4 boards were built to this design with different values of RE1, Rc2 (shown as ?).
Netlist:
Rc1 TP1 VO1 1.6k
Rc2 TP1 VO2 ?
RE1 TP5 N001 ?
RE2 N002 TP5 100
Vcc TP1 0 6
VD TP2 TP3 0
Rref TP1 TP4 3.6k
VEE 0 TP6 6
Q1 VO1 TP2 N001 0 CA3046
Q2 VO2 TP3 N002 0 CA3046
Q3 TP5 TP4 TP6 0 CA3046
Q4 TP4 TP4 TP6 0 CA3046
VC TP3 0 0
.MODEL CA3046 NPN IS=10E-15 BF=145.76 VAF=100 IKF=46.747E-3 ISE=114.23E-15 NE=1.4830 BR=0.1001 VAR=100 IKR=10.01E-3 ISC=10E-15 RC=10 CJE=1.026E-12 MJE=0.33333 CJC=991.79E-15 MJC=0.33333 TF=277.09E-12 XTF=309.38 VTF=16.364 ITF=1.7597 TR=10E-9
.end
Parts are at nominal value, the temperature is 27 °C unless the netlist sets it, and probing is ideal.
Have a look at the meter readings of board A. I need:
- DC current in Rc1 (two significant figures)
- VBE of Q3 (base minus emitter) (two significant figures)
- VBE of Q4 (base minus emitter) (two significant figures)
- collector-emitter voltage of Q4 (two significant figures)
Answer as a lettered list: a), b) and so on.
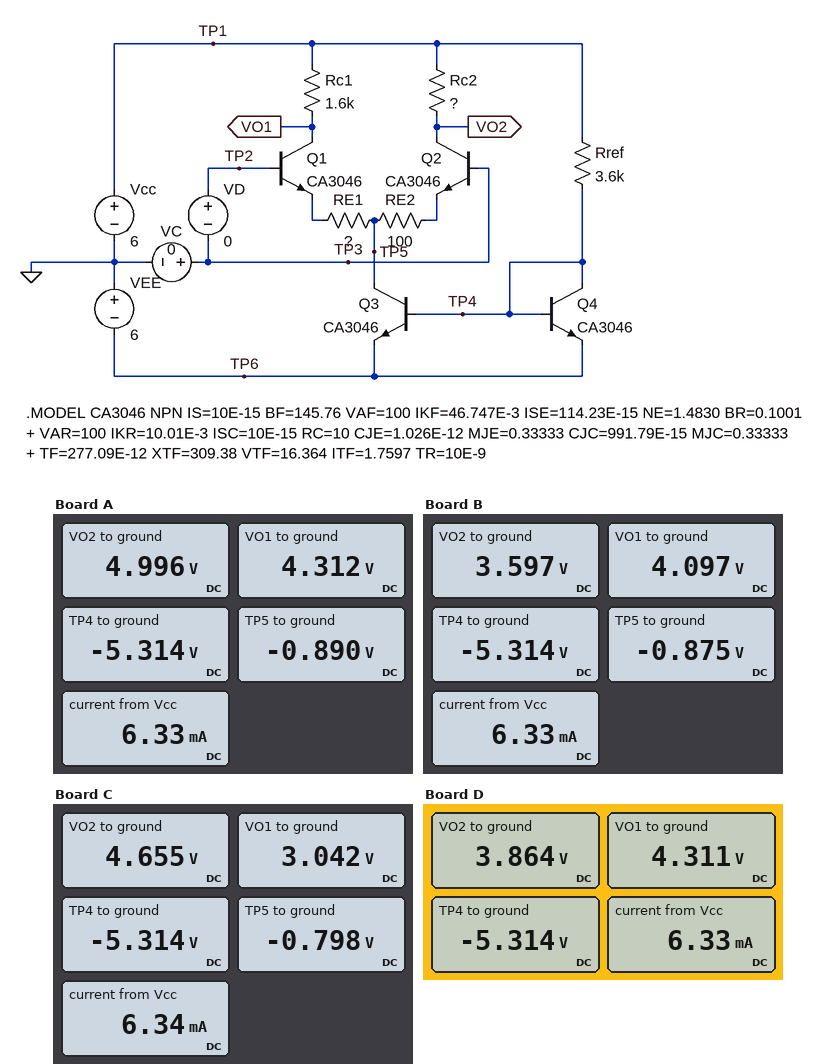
a) 1.1 mA
b) 690 mV
c) 690 mV
d) 690 mV
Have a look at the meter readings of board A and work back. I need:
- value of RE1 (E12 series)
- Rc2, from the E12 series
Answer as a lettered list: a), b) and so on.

a) 220 Ω
b) 470 Ω
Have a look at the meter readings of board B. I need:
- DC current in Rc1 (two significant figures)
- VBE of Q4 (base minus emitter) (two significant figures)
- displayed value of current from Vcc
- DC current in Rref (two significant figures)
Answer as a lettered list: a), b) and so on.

a) 1.2 mA
b) 690 mV
c) 6.33 mA
d) 3.1 mA
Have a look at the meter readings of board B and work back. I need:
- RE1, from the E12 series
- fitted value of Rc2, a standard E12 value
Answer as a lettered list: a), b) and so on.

a) 180 Ω
b) 1.2 kΩ
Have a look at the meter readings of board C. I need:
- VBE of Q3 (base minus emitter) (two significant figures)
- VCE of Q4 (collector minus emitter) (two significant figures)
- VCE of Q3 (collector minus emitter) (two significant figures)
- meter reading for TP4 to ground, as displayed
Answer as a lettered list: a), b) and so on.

a) 690 mV
b) 690 mV
c) 5.2 V
d) -5.314 V
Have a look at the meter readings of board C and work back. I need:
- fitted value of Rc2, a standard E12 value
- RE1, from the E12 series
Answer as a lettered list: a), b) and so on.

a) 1 kΩ
b) 68 Ω
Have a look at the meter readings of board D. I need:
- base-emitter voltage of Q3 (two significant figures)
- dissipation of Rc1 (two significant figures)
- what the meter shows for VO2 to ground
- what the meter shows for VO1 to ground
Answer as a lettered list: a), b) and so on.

a) 690 mV
b) 1.8 mW
c) 3.864 V
d) 4.311 V
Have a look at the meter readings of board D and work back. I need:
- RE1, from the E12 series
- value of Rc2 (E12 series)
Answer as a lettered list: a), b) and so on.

a) 220 Ω
b) 1 kΩ
